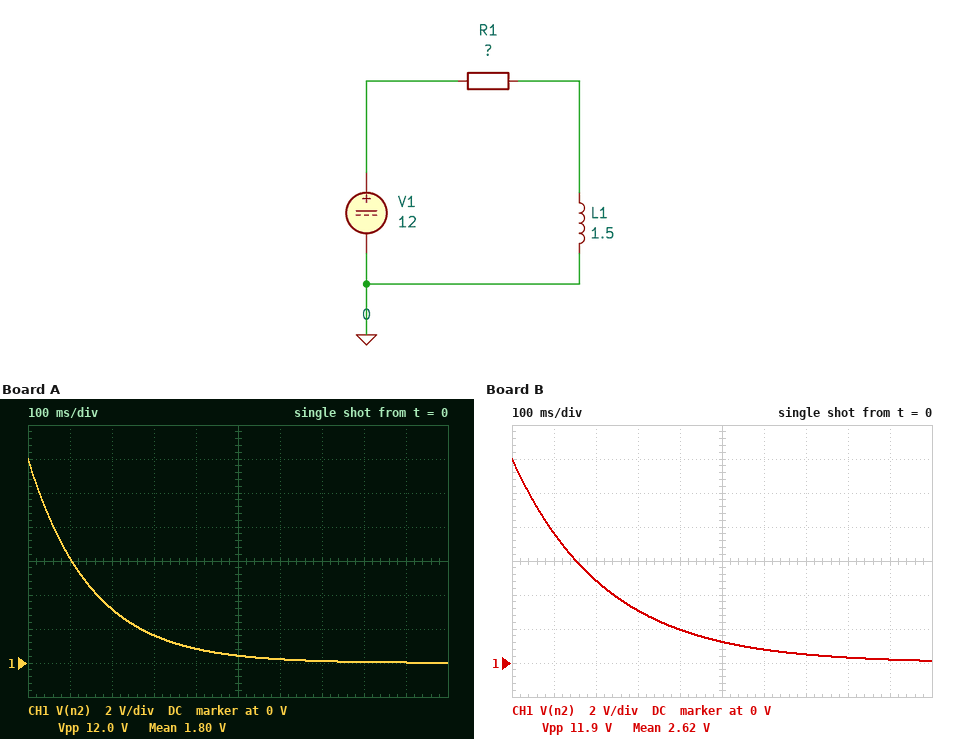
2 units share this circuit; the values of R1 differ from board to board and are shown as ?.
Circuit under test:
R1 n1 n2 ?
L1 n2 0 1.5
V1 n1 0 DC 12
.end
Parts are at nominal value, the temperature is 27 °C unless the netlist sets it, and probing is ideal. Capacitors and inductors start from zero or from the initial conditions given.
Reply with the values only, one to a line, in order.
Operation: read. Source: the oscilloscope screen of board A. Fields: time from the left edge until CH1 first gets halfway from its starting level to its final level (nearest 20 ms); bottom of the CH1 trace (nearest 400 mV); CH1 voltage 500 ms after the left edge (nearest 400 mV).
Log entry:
100 ms
0 V
400 mV
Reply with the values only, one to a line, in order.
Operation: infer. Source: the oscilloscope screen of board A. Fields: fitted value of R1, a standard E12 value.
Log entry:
10 Ω
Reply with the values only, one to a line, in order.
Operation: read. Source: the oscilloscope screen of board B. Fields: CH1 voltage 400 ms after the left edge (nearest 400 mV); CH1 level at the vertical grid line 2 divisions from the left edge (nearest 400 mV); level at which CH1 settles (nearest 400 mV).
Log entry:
2.0 V
4.8 V
0 V
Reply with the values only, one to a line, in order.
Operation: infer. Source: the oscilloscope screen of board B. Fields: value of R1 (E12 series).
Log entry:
6.8 Ω
